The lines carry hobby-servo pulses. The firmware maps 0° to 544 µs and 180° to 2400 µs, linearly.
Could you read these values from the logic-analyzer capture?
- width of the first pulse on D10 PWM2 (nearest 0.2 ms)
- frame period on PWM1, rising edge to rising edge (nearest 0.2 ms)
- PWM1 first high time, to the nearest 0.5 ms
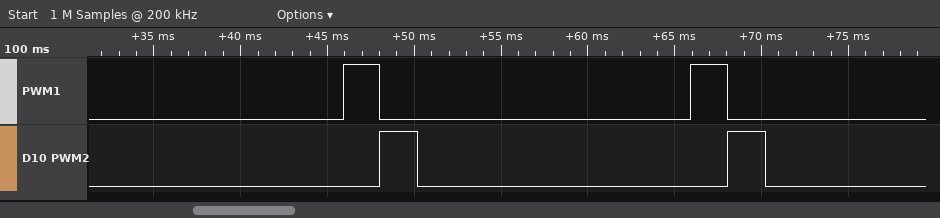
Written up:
2.2 ms
20.0 ms
2.0 ms
